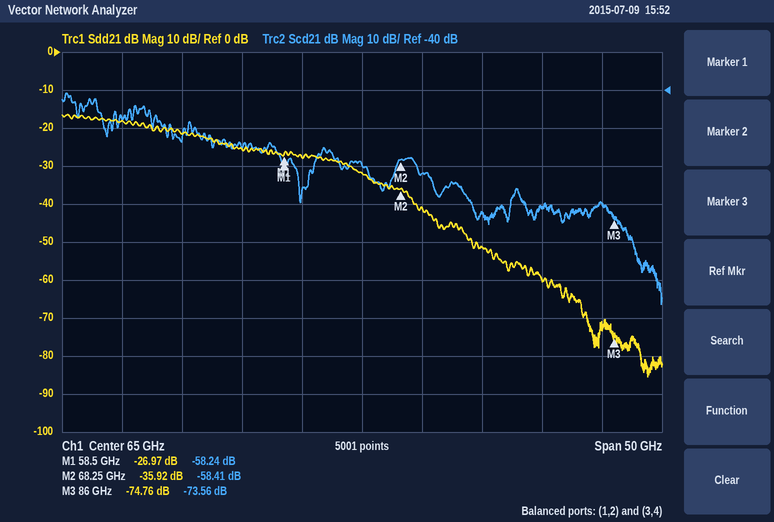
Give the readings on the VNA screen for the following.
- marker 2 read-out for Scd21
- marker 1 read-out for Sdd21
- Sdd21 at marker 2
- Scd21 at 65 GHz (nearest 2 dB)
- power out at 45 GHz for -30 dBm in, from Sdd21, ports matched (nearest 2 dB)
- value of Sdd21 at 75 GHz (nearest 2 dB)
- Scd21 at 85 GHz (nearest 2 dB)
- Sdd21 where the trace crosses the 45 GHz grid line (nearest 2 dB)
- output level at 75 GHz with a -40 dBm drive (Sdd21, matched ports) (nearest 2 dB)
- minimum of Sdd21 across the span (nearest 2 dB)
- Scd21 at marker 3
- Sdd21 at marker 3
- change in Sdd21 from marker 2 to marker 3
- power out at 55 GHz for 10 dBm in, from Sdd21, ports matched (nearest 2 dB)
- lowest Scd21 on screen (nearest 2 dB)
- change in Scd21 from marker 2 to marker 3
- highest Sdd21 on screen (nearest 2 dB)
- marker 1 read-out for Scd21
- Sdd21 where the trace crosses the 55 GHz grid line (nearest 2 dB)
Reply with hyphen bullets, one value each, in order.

- -58.41 dB
- -26.97 dB
- -35.92 dB
- -60 dB
- -48 dBm
- -52 dB
- -70 dB
- -18 dB
- -92 dBm
- -86 dB
- -73.56 dB
- -74.76 dB
- -38.84 dB
- -16 dBm
- -96 dB
- -15.15 dB
- -16 dB
- -58.24 dB
- -26 dB
